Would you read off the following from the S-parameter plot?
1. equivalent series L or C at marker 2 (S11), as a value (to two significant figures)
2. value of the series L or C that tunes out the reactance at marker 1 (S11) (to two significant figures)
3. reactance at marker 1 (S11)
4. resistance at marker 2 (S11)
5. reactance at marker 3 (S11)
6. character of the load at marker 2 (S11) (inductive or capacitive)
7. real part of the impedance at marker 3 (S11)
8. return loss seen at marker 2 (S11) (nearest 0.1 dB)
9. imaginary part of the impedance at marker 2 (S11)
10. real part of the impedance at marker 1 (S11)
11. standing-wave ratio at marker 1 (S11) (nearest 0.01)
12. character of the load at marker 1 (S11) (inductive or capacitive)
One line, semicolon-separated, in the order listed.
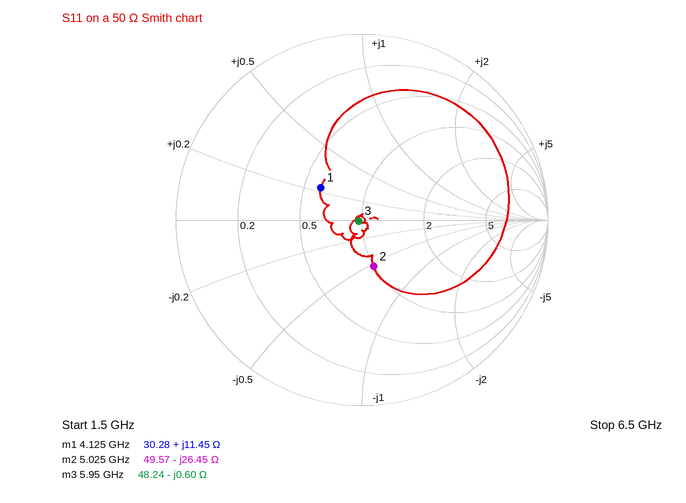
1.2 pF; 3.4 pF; +11.45 Ω; 49.57 Ω; -0.60 Ω; capacitive; 48.24 Ω; 11.8 dB; -26.45 Ω; 30.28 Ω; 1.78; inductive
